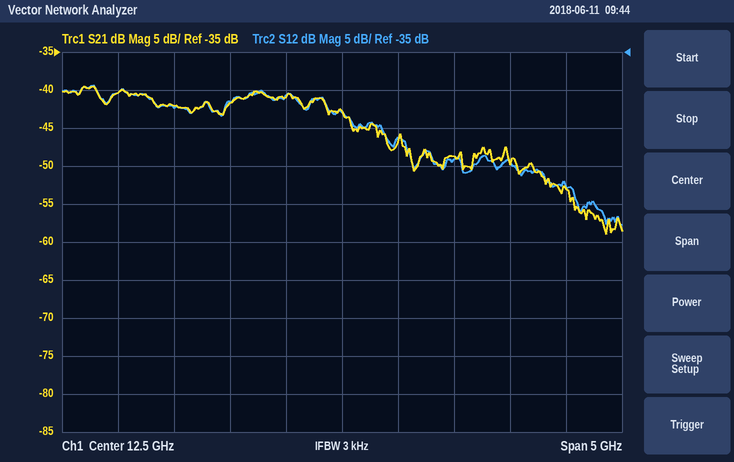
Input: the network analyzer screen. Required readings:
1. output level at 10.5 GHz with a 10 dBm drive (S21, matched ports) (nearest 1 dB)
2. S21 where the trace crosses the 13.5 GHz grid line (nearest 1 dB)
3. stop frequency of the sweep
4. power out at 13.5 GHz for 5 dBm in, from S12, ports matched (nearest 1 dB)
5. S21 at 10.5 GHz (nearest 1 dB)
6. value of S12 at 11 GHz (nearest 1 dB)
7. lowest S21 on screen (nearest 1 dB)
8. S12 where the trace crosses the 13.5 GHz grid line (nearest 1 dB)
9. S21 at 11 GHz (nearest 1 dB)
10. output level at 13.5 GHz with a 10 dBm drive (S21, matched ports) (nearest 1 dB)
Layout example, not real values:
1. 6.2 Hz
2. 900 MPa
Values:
1. -30 dBm
2. -49 dB
3. 15 GHz
4. -44 dBm
5. -40 dB
6. -42 dB
7. -59 dB
8. -49 dB
9. -42 dB
10. -39 dBm
